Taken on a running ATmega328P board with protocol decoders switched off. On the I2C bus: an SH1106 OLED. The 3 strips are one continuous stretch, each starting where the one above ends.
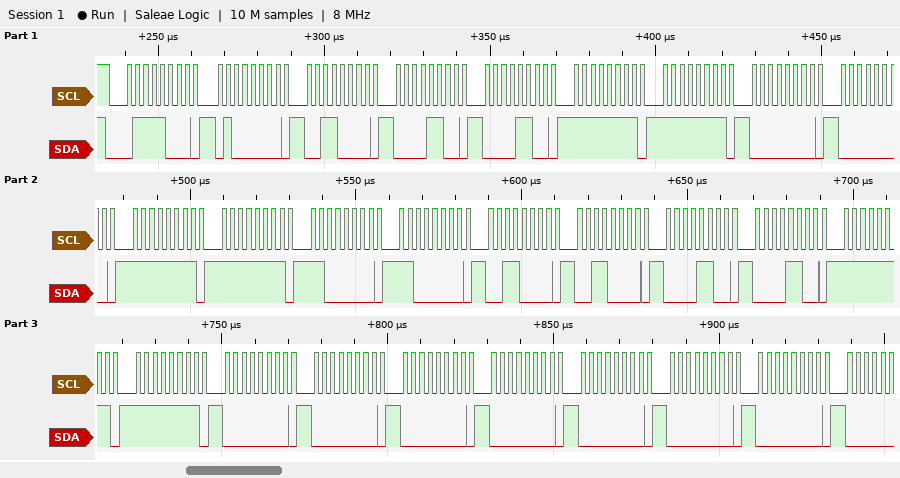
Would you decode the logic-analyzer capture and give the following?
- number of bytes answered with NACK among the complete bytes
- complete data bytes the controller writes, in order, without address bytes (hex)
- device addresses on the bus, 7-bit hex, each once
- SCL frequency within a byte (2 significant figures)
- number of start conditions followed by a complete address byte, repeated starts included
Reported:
0
40 30 0C 0C FF FF 00 00 FF FF C0 C0 30 30 0C 0C FF FF 00 00 00 00 00 00 00
0x3C
400 kHz
1
